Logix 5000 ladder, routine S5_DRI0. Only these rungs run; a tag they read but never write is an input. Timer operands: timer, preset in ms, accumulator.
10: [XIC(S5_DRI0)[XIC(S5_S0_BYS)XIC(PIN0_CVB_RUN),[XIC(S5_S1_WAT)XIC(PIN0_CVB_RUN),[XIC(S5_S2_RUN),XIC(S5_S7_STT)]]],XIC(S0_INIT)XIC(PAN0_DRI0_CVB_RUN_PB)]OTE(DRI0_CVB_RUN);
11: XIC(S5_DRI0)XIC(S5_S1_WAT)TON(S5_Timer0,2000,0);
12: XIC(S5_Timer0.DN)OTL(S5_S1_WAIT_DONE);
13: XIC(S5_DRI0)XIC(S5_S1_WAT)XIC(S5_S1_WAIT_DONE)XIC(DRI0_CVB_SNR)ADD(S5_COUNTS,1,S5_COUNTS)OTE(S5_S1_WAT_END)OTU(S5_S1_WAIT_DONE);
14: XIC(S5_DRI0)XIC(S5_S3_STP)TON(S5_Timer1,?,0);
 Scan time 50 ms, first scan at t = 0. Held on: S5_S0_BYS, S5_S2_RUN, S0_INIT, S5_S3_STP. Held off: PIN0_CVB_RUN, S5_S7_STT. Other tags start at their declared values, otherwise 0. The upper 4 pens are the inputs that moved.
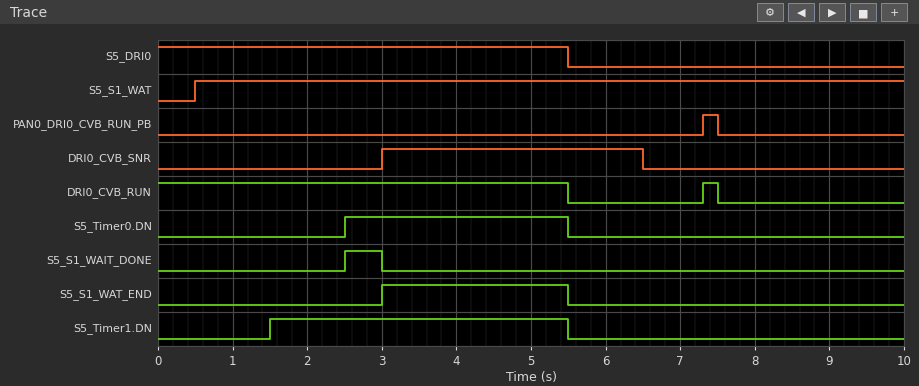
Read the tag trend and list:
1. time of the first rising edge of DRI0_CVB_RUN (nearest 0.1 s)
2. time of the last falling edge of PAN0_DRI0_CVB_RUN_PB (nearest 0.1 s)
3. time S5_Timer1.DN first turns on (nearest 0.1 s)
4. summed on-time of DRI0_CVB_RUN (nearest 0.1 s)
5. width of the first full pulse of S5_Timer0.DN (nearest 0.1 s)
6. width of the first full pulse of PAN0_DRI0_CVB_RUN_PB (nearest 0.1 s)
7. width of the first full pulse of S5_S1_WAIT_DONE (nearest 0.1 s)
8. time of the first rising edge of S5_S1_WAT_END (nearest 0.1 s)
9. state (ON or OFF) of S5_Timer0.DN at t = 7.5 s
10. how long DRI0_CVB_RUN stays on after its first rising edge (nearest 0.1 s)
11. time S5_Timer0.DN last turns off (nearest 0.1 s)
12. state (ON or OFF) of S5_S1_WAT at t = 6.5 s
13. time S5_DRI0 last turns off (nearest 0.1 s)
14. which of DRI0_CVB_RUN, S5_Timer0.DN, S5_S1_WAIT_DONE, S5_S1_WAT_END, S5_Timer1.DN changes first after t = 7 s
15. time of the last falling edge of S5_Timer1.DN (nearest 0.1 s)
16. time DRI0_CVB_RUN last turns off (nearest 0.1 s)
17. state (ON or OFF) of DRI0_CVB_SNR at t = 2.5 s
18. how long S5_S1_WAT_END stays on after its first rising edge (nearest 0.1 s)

7.3 s
7.5 s
1.5 s
5.7 s
3.0 s
0.2 s
0.5 s
3.0 s
OFF
0.2 s
5.5 s
ON
5.5 s
DRI0_CVB_RUN
5.5 s
7.5 s
OFF
2.5 s
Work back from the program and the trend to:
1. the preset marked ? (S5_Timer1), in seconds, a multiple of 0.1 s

1.5 s
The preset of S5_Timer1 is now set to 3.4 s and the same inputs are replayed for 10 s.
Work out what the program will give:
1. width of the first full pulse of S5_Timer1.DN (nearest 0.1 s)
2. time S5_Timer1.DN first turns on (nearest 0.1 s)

2.1 s
3.4 s
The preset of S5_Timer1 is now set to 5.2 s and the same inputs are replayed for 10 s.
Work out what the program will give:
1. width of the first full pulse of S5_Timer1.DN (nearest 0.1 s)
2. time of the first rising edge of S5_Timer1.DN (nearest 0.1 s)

0.3 s
5.2 s
